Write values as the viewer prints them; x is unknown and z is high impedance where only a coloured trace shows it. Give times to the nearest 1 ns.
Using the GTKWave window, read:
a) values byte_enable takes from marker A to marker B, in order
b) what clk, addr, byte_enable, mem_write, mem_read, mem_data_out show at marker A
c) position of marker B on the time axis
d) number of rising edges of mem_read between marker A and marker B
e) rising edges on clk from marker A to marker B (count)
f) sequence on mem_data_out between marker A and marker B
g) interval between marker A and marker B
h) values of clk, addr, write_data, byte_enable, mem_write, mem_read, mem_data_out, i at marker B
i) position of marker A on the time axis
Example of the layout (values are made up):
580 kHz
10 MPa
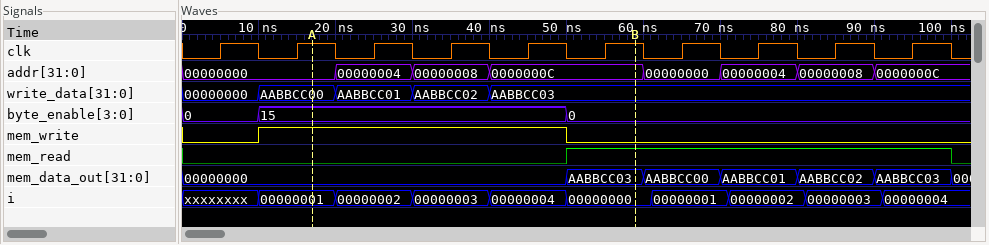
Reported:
15, 0
clk=1, addr=00000000, byte_enable=15, mem_write=1, mem_read=0, mem_data_out=00000000
59 ns
1
4
00000000, AABBCC03
42 ns
clk=1, addr=0000000C, write_data=AABBCC03, byte_enable=0, mem_write=0, mem_read=1, mem_data_out=AABBCC03, i=00000000
17 ns
